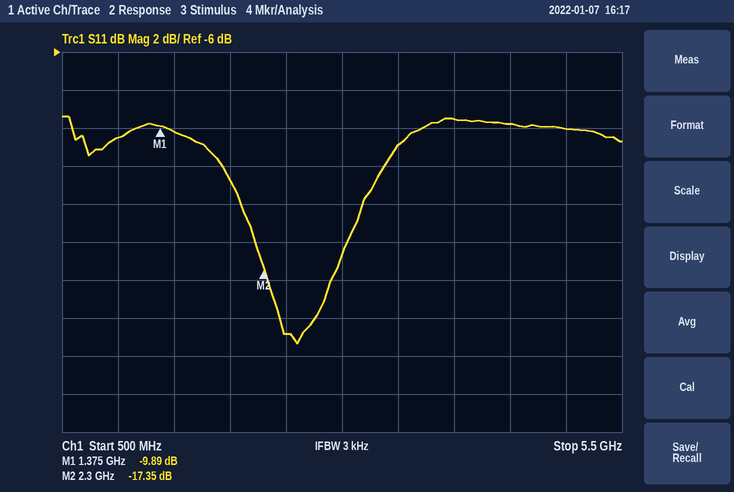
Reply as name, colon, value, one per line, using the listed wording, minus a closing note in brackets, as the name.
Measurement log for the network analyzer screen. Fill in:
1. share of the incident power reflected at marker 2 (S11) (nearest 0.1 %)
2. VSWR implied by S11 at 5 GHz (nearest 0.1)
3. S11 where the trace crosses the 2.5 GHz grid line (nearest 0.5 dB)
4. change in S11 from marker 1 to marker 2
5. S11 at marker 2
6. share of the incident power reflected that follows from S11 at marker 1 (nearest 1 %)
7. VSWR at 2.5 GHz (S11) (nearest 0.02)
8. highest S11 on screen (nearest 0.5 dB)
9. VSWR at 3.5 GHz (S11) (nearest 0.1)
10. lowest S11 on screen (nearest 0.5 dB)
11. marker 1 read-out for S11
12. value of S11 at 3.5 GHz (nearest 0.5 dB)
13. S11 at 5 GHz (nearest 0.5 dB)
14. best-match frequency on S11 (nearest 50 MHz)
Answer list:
share of the incident power reflected at marker 2 (S11): 1.8 %
VSWR implied by S11 at 5 GHz: 1.9
S11 where the trace crosses the 2.5 GHz grid line: -21.0 dB
change in S11 from marker 1 to marker 2: -7.46 dB
S11 at marker 2: -17.35 dB
share of the incident power reflected that follows from S11 at marker 1: 10 %
VSWR at 2.5 GHz (S11): 1.20
highest S11 on screen: -9.5 dB
VSWR at 3.5 GHz (S11): 1.8
lowest S11 on screen: -21.5 dB
marker 1 read-out for S11: -9.89 dB
value of S11 at 3.5 GHz: -11.0 dB
S11 at 5 GHz: -10.0 dB
best-match frequency on S11: 2.60 GHz
